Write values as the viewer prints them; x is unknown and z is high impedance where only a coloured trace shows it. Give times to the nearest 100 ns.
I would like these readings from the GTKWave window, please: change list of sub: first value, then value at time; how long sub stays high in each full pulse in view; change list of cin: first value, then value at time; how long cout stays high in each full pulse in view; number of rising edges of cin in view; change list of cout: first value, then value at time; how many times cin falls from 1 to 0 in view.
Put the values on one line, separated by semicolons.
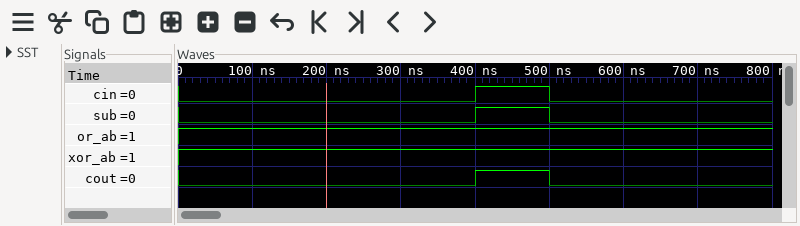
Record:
0, 1 at 400 ns, 0 at 500 ns; 100 ns; 0, 1 at 400 ns, 0 at 500 ns; 100 ns; 1; 0, 1 at 400 ns, 0 at 500 ns; 1
